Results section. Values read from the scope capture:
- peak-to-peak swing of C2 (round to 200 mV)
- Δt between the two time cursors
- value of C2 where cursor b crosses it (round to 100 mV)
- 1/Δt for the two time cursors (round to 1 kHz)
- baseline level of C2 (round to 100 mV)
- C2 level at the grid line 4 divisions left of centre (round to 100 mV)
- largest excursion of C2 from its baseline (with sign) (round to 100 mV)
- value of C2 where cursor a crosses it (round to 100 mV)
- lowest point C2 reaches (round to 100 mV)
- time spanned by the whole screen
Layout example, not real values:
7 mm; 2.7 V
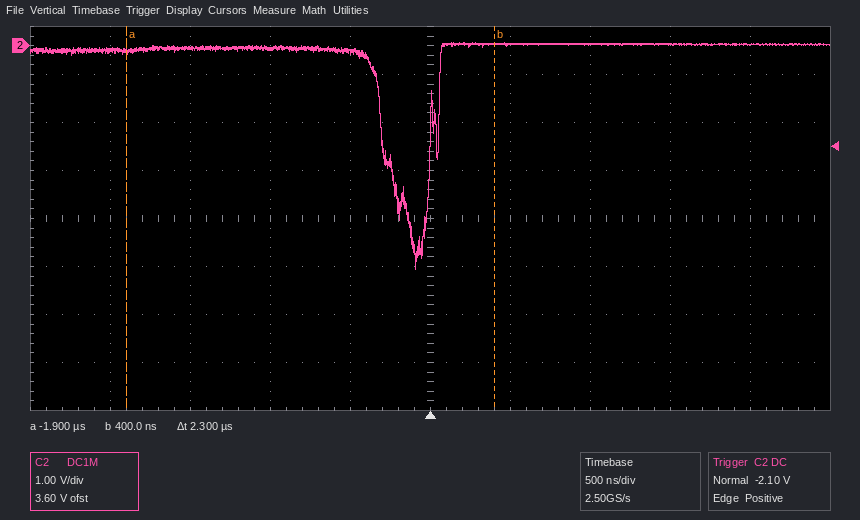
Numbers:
4.8 V; 2.3 µs; 0.0 V; 435 kHz; 0.0 V; -100 mV; -4.7 V; -100 mV; -4.7 V; 5 µs
